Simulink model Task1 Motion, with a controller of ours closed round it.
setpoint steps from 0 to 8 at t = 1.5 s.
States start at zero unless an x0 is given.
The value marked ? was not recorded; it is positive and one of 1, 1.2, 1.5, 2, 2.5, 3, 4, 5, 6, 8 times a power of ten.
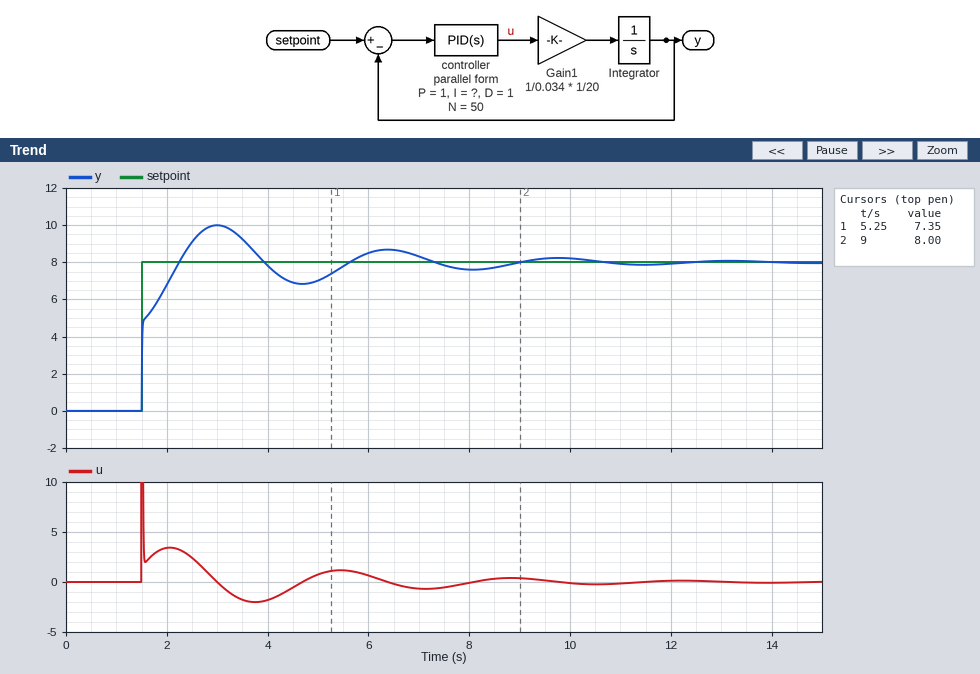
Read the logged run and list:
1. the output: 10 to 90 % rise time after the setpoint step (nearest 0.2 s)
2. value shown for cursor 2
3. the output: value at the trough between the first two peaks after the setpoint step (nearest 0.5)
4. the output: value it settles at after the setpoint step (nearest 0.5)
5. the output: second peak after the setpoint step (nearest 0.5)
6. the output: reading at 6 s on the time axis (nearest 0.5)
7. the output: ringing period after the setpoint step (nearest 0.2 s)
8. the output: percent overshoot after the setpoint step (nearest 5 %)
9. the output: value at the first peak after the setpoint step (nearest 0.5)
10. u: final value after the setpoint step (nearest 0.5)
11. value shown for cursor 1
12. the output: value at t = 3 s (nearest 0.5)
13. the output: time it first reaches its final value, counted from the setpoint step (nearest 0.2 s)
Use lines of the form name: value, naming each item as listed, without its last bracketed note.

the output: 10 to 90 % rise time after the setpoint step: 0.6 s
value shown for cursor 2: 8.00
the output: value at the trough between the first two peaks after the setpoint step: 7.0
the output: value it settles at after the setpoint step: 8.0
the output: second peak after the setpoint step: 8.5
the output: reading at 6 s on the time axis: 8.5
the output: ringing period after the setpoint step: 3.4 s
the output: percent overshoot after the setpoint step: 25 %
the output: value at the first peak after the setpoint step: 10.0
u: final value after the setpoint step: 0.0
value shown for cursor 1: 7.35
the output: value at t = 3 s: 10.0
the output: time it first reaches its final value, counted from the setpoint step: 0.8 s
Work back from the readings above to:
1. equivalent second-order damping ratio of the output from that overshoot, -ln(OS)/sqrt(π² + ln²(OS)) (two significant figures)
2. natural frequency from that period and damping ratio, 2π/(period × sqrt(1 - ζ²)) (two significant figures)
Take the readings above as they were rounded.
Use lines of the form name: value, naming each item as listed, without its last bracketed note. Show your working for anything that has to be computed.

equivalent second-order damping ratio of the output from that overshoot, -ln(OS)/sqrt(π² + ln²(OS)): ln(0.25) = -1.386; 1.386 / sqrt(9.870 + 1.922) = 0.40
natural frequency from that period and damping ratio, 2π/(period × sqrt(1 - ζ²)): 2π / (3.4 × sqrt(1 - 0.4²)) = 2.0 rad/s
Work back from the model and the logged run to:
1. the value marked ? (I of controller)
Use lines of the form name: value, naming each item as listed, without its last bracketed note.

the value marked ?: 6
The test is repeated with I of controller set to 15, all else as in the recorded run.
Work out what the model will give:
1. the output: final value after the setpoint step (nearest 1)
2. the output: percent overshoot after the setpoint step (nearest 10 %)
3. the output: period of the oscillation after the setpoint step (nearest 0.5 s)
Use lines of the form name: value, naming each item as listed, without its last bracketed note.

the output: final value after the setpoint step: 8
the output: percent overshoot after the setpoint step: 30 %
the output: period of the oscillation after the setpoint step: 2.0 s
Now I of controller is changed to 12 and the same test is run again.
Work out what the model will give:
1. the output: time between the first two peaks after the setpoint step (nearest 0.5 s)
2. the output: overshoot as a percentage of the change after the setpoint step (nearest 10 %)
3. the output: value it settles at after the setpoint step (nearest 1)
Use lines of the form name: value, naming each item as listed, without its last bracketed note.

the output: time between the first two peaks after the setpoint step: 2.5 s
the output: overshoot as a percentage of the change after the setpoint step: 30 %
the output: value it settles at after the setpoint step: 8
